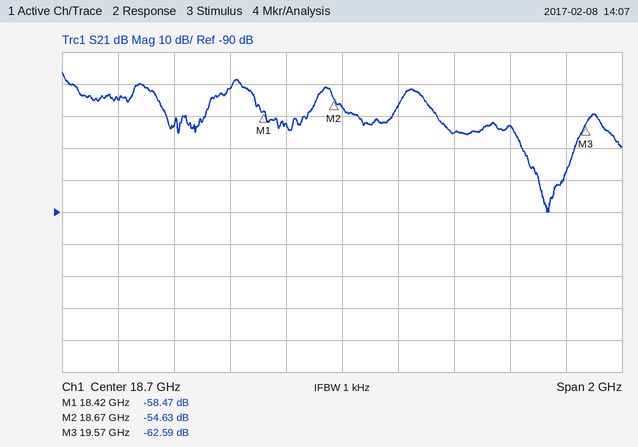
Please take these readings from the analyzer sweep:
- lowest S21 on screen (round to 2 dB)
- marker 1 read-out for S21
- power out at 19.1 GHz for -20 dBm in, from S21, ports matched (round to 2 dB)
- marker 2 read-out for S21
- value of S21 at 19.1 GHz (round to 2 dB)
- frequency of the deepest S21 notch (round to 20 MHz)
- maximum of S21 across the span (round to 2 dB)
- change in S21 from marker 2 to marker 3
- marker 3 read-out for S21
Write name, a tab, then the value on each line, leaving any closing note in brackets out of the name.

lowest S21 on screen	-90 dB
marker 1 read-out for S21	-58.47 dB
power out at 19.1 GHz for -20 dBm in, from S21, ports matched	-86 dBm
marker 2 read-out for S21	-54.63 dB
value of S21 at 19.1 GHz	-66 dB
frequency of the deepest S21 notch	19.44 GHz
maximum of S21 across the span	-46 dB
change in S21 from marker 2 to marker 3	-7.96 dB
marker 3 read-out for S21	-62.59 dB
